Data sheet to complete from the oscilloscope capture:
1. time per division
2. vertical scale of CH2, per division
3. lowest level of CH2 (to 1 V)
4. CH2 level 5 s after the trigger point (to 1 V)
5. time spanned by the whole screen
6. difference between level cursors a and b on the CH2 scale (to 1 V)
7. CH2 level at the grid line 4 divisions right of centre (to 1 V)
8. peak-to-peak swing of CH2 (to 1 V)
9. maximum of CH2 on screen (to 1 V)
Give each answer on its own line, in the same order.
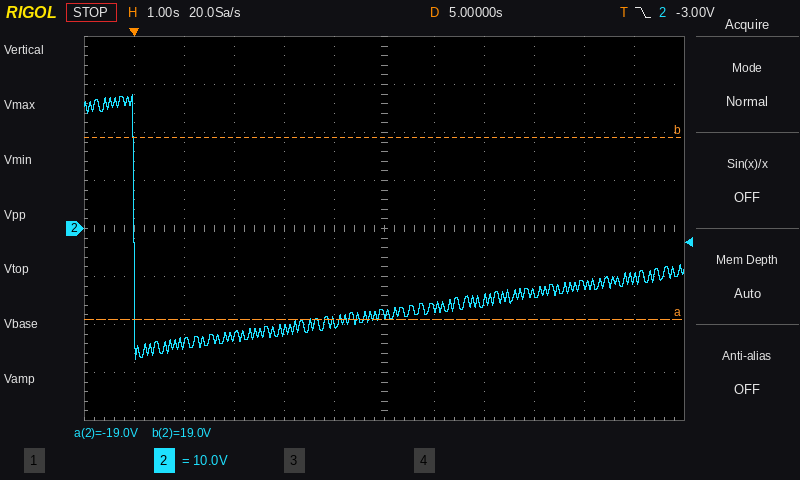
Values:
1 s
10 V
-27 V
-18 V
12 s
38 V
-12 V
55 V
28 V
